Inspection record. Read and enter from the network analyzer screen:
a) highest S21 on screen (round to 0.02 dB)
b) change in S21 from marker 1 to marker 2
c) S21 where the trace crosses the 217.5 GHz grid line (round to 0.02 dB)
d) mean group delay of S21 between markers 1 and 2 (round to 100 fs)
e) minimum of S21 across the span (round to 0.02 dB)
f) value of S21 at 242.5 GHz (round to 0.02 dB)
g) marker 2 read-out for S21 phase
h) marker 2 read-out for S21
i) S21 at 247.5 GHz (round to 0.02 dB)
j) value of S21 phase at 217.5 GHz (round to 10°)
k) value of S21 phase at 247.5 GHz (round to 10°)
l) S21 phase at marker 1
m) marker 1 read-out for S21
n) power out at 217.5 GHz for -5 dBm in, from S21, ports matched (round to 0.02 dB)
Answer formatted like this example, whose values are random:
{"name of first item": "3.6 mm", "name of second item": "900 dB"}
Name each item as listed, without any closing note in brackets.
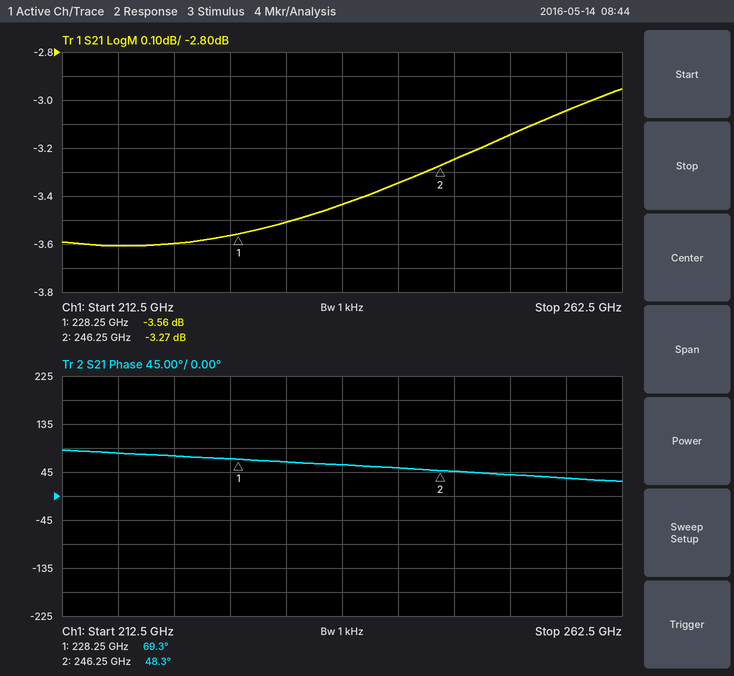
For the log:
{"highest S21 on screen": "-2.96 dB", "change in S21 from marker 1 to marker 2": "0.29 dB", "S21 where the trace crosses the 217.5 GHz grid line": "-3.60 dB", "mean group delay of S21 between markers 1 and 2": "3.2 ps", "minimum of S21 across the span": "-3.60 dB", "value of S21 at 242.5 GHz": "-3.34 dB", "marker 2 read-out for S21 phase": "48.3°", "marker 2 read-out for S21": "-3.27 dB", "S21 at 247.5 GHz": "-3.24 dB", "value of S21 phase at 217.5 GHz": "80°", "value of S21 phase at 247.5 GHz": "50°", "S21 phase at marker 1": "69.3°", "marker 1 read-out for S21": "-3.56 dB", "power out at 217.5 GHz for -5 dBm in, from S21, ports matched": "-8.60 dBm"}
